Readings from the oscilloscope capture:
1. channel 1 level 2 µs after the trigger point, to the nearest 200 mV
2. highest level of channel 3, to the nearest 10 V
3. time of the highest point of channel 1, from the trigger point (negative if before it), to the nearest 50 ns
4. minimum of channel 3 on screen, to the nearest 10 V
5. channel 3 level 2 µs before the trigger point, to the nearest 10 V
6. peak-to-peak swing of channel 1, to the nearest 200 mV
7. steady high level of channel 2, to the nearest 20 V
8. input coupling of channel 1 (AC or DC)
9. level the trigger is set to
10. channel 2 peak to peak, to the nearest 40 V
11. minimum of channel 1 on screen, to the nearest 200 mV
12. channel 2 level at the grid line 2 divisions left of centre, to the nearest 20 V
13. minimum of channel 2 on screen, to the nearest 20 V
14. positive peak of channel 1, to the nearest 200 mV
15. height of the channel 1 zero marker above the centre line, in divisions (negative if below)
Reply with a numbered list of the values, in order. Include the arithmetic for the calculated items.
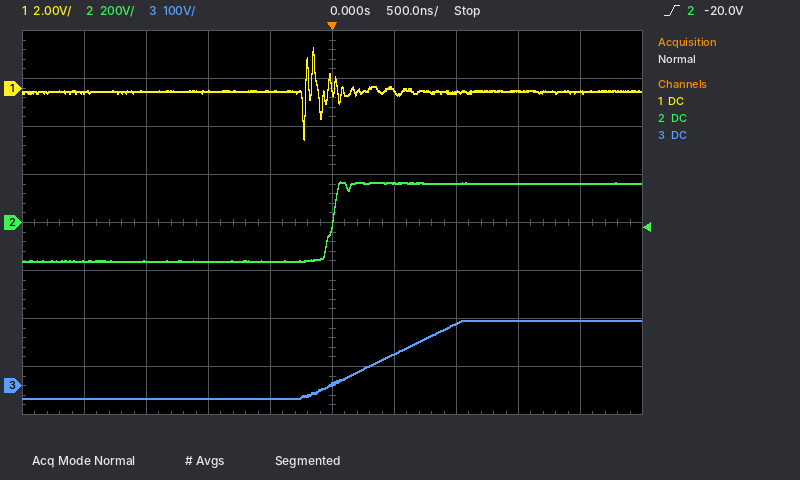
1. -200 mV
2. 140 V
3. -150 ns
4. -30 V
5. -30 V
6. 1.6 V − (-2.2 V) = 3.8 V
7. 160 V
8. DC
9. -20.0 V
10. 320 V
11. -2.2 V
12. -160 V
13. -160 V
14. 1.6 V
15. +2.8 div
